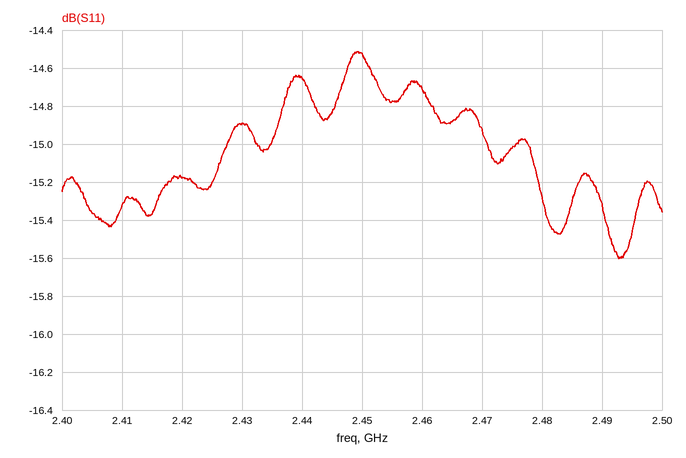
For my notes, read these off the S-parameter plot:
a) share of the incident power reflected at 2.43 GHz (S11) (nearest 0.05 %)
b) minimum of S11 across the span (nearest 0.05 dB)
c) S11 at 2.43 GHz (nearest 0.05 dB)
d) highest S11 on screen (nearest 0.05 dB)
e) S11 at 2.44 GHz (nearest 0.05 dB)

3.25 %
-15.60 dB
-14.90 dB
-14.50 dB
-14.65 dB
